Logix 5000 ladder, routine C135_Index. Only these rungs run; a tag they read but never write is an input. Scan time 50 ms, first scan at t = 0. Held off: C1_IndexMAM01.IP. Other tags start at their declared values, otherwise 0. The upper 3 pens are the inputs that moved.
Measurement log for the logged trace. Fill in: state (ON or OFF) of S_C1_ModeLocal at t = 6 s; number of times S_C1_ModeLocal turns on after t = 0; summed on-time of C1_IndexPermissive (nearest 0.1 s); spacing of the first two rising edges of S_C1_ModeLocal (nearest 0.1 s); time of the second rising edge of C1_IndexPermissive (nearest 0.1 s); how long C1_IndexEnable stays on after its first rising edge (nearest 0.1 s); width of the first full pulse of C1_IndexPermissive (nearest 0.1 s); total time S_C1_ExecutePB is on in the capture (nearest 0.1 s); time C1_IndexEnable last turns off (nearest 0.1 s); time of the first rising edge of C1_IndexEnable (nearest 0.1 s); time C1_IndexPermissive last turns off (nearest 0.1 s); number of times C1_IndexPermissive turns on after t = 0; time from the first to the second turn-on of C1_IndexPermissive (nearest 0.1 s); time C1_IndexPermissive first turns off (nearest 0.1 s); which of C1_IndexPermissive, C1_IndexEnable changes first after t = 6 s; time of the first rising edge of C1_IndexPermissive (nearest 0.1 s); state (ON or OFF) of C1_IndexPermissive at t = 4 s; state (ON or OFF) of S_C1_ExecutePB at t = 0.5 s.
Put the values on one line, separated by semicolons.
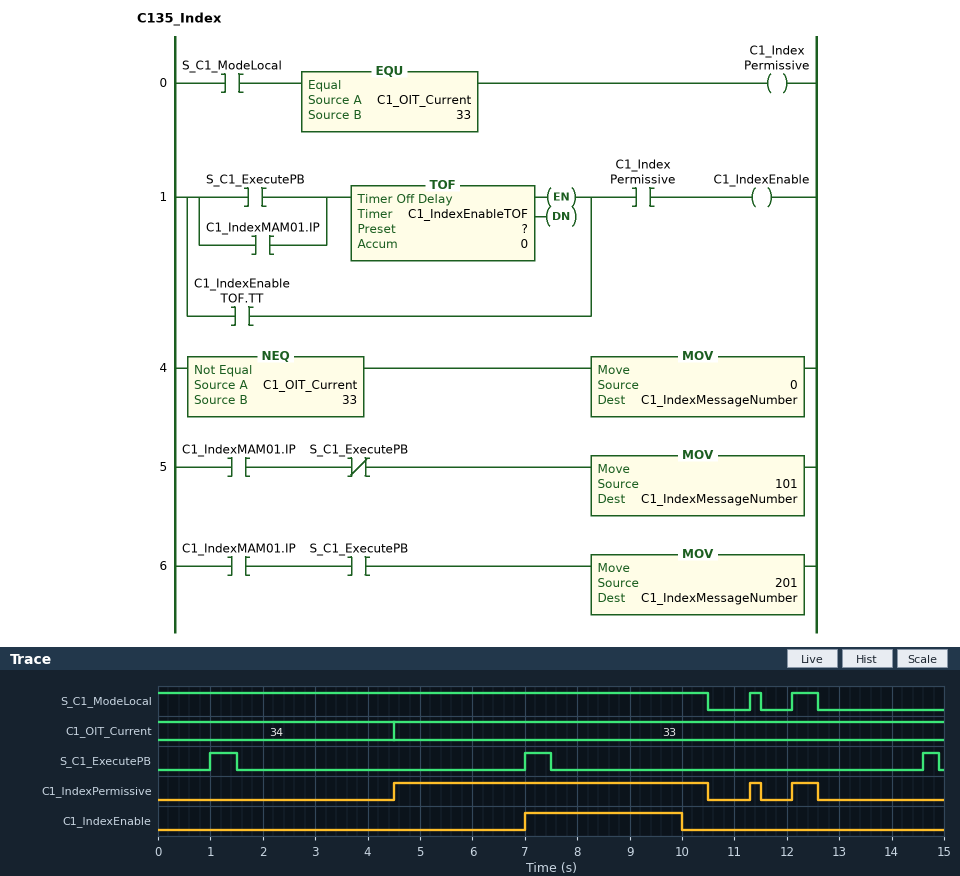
ON; 2; 6.7 s; 0.8 s; 11.3 s; 3.0 s; 6.0 s; 1.3 s; 10.0 s; 7.0 s; 12.6 s; 3; 6.8 s; 10.5 s; C1_IndexEnable; 4.5 s; OFF; OFF
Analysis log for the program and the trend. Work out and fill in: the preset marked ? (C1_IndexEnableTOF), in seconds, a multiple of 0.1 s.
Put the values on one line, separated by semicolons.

2.5 s
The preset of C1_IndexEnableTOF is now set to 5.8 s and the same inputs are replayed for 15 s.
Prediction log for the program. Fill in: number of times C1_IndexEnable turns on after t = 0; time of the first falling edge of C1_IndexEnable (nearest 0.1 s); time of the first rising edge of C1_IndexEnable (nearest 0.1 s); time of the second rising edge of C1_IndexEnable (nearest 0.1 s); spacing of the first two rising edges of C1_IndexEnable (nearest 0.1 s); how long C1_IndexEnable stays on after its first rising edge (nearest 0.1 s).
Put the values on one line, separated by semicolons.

3; 10.5 s; 4.5 s; 11.3 s; 6.8 s; 6.0 s
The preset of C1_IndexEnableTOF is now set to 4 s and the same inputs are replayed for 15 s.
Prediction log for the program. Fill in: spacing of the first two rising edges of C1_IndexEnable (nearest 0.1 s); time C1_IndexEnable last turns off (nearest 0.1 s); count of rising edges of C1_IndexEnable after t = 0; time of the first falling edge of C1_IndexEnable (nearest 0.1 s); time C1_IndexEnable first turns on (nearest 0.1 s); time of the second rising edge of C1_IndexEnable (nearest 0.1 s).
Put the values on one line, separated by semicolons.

2.5 s; 11.5 s; 3; 5.5 s; 4.5 s; 7.0 s
